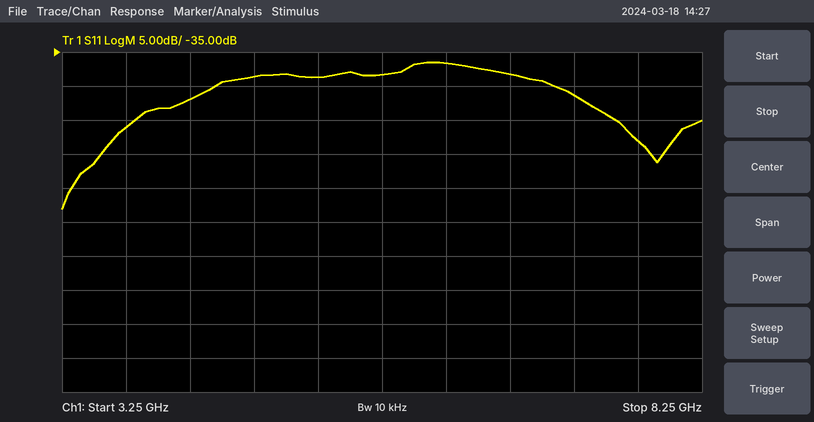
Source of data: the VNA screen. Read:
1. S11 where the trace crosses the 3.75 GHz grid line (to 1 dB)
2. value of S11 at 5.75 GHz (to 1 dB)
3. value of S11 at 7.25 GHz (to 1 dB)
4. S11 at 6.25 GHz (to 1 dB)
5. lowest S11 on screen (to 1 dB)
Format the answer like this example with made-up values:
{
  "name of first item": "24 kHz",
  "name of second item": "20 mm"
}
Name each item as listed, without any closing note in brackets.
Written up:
{
  "S11 where the trace crosses the 3.75 GHz grid line": "-46 dB",
  "value of S11 at 5.75 GHz": "-38 dB",
  "value of S11 at 7.25 GHz": "-41 dB",
  "S11 at 6.25 GHz": "-37 dB",
  "lowest S11 on screen": "-58 dB"
}
